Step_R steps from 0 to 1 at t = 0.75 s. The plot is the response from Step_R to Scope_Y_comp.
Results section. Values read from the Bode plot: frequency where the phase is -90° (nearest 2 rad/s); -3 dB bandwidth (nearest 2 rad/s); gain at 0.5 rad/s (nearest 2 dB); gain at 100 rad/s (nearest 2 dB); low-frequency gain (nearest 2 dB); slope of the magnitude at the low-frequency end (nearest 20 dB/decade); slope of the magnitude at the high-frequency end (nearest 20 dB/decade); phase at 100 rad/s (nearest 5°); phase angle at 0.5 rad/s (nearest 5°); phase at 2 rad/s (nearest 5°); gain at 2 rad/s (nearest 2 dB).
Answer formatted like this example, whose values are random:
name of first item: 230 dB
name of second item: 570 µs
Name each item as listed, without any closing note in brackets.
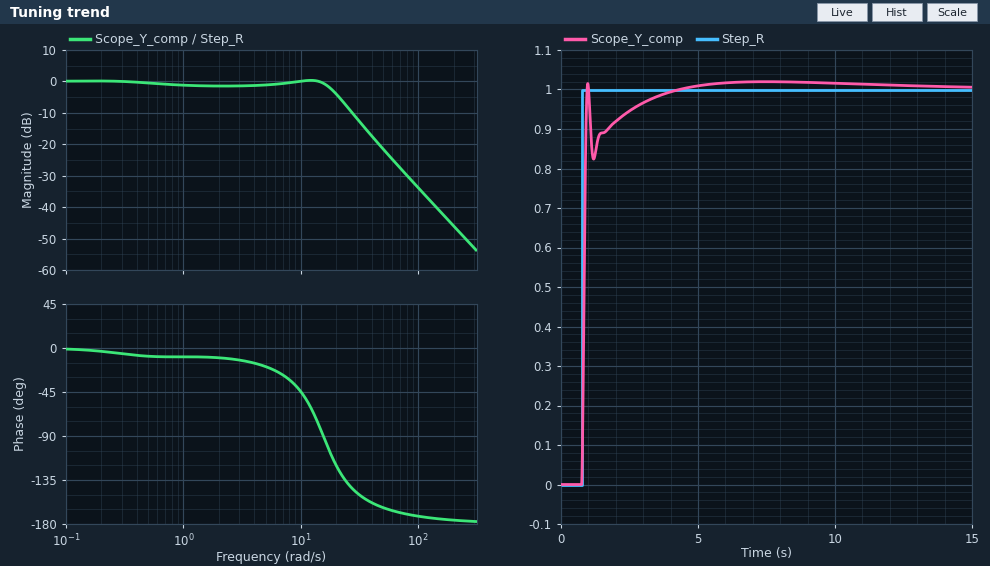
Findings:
frequency where the phase is -90°: 16 rad/s
-3 dB bandwidth: 18 rad/s
gain at 0.5 rad/s: 0 dB
gain at 100 rad/s: -34 dB
low-frequency gain: 0 dB
slope of the magnitude at the low-frequency end: 0 dB/decade
slope of the magnitude at the high-frequency end: -40 dB/decade
phase at 100 rad/s: -170°
phase angle at 0.5 rad/s: -10°
phase at 2 rad/s: -10°
gain at 2 rad/s: -2 dB
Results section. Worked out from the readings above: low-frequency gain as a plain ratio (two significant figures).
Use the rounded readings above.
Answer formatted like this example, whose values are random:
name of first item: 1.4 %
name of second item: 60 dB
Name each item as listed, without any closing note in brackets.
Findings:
low-frequency gain as a plain ratio: 1.0
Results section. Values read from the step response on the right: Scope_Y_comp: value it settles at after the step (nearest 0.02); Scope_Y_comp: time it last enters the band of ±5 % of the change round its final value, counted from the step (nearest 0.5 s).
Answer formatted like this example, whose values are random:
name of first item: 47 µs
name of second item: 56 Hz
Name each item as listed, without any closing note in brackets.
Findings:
Scope_Y_comp: value it settles at after the step: 1.00
Scope_Y_comp: time it last enters the band of ±5 % of the change round its final value, counted from the step: 2.0 s
